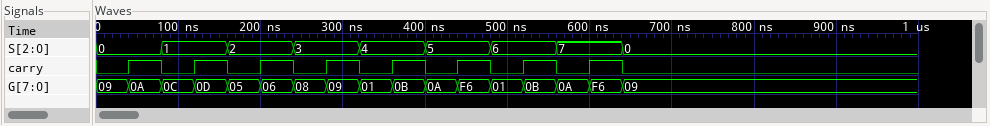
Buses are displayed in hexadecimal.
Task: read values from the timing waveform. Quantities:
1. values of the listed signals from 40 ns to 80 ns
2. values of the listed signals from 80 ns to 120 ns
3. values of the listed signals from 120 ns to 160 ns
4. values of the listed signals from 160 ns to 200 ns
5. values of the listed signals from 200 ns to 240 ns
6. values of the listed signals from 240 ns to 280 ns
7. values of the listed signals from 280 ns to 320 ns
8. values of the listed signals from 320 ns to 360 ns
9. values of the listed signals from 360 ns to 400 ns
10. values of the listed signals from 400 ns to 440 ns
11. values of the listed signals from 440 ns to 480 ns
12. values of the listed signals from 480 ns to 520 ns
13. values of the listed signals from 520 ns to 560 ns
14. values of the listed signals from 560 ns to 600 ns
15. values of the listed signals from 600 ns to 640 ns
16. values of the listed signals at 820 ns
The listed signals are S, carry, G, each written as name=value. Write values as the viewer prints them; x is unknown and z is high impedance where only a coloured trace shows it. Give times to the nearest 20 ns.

S=0, carry=1, G=0A
S=1, carry=0, G=0C
S=1, carry=1, G=0D
S=2, carry=0, G=05
S=2, carry=1, G=06
S=3, carry=0, G=08
S=3, carry=1, G=09
S=4, carry=0, G=01
S=4, carry=1, G=0B
S=5, carry=0, G=0A
S=5, carry=1, G=F6
S=6, carry=0, G=01
S=6, carry=1, G=0B
S=7, carry=0, G=0A
S=7, carry=1, G=F6
S=0, carry=0, G=09
